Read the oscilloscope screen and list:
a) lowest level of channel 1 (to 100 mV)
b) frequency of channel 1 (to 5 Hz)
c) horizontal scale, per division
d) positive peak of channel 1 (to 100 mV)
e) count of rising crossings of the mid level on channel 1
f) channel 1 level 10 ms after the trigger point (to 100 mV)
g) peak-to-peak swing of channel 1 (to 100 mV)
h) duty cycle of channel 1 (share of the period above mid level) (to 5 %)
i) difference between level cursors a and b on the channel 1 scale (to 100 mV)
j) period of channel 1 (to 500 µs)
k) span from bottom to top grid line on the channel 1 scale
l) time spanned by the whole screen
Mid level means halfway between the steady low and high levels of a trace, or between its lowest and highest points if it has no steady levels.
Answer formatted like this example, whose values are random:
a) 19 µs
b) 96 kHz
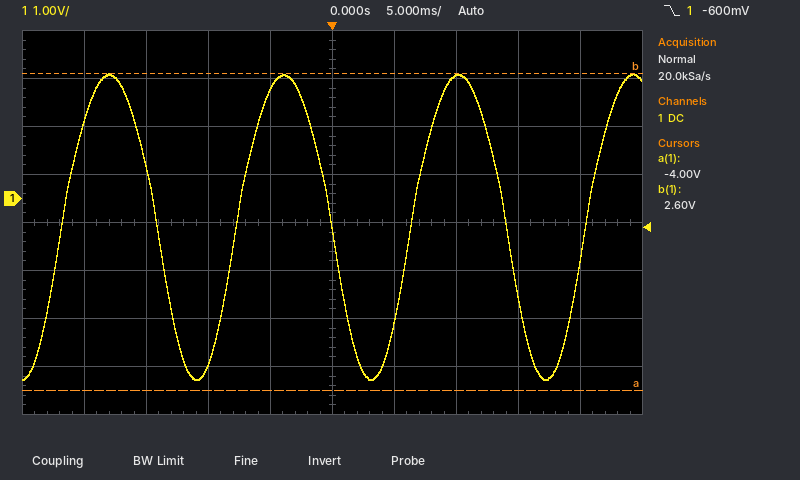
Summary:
a) -3.8 V
b) 70 Hz
c) 5 ms
d) 2.6 V
e) 4
f) 2.6 V
g) 6.4 V
h) 55 %
i) 6.6 V
j) 14.0 ms
k) 8 V
l) 50 ms
